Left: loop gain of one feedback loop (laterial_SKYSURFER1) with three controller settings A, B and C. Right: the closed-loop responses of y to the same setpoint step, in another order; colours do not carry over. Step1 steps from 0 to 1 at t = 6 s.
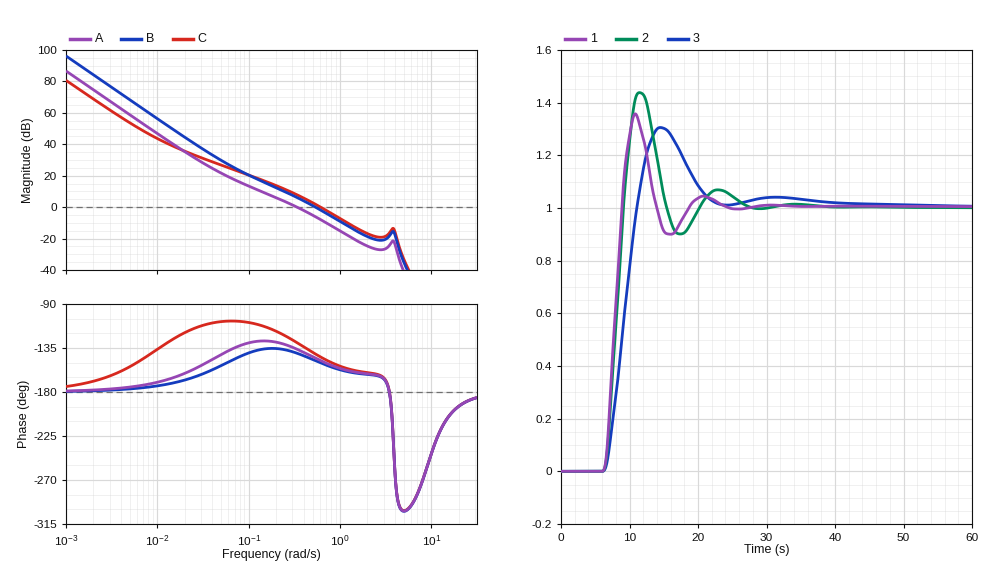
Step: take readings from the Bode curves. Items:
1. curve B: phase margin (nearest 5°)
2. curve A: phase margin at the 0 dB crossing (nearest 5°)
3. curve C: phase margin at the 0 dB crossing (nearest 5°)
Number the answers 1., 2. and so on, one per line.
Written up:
1. 30°
2. 45°
3. 35°
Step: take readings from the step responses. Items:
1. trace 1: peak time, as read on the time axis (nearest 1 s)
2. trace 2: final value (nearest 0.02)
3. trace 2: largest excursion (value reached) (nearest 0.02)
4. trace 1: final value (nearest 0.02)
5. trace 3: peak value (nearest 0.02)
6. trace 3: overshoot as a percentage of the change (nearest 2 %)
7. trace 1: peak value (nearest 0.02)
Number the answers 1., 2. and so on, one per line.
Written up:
1. 11 s
2. 1.00
3. 1.44
4. 1.00
5. 1.30
6. 30 %
7. 1.36
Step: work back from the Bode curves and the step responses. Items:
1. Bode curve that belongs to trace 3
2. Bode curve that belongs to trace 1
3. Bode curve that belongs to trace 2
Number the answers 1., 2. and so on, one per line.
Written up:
1. A
2. C
3. B
